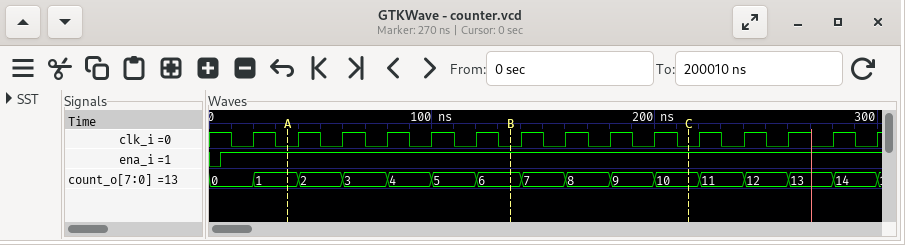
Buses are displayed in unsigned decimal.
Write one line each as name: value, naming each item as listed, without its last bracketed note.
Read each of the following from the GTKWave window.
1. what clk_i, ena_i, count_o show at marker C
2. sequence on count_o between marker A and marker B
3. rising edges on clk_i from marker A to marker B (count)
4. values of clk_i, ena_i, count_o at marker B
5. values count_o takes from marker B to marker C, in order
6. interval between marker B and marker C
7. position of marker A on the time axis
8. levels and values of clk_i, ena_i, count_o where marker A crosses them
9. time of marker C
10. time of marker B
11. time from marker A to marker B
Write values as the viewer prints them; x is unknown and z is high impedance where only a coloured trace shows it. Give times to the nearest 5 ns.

what clk_i, ena_i, count_o show at marker C: clk_i=0, ena_i=1, count_o=10
sequence on count_o between marker A and marker B: 1, 2, 3, 4, 5, 6
rising edges on clk_i from marker A to marker B: 5
values of clk_i, ena_i, count_o at marker B: clk_i=0, ena_i=1, count_o=6
values count_o takes from marker B to marker C, in order: 6, 7, 8, 9, 10
interval between marker B and marker C: 80 ns
position of marker A on the time axis: 35 ns
levels and values of clk_i, ena_i, count_o where marker A crosses them: clk_i=0, ena_i=1, count_o=1
time of marker C: 215 ns
time of marker B: 135 ns
time from marker A to marker B: 100 ns
